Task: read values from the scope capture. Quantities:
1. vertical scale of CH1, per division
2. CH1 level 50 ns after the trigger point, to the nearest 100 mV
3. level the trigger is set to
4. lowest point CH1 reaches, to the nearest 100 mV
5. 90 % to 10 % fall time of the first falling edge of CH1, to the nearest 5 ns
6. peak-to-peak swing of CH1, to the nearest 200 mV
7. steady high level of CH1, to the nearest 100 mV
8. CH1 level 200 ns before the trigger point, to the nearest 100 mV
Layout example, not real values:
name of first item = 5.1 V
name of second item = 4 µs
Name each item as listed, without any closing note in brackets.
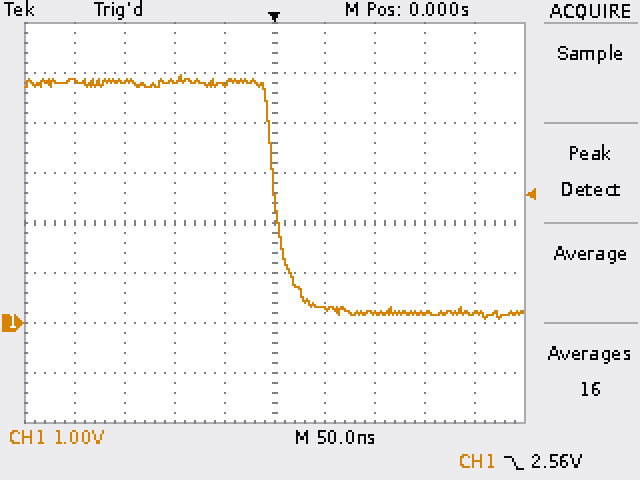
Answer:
vertical scale of CH1, per division = 1 V
CH1 level 50 ns after the trigger point, to the nearest 100 mV = 300 mV
level the trigger is set to = 2.56 V
lowest point CH1 reaches, to the nearest 100 mV = 100 mV
90 % to 10 % fall time of the first falling edge of CH1, to the nearest 5 ns = 35 ns
peak-to-peak swing of CH1, to the nearest 200 mV = 4.8 V
steady high level of CH1, to the nearest 100 mV = 4.8 V
CH1 level 200 ns before the trigger point, to the nearest 100 mV = 4.8 V
